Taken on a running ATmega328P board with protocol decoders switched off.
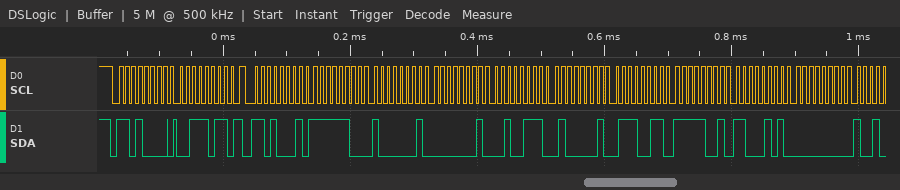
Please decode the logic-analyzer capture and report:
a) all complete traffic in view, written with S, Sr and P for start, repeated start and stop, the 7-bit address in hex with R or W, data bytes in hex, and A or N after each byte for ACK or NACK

S 68W A 3B A Sr 68R A FC A 81 A 01 A 27 A 41 A 73 A F9 A C5 A 00 A
